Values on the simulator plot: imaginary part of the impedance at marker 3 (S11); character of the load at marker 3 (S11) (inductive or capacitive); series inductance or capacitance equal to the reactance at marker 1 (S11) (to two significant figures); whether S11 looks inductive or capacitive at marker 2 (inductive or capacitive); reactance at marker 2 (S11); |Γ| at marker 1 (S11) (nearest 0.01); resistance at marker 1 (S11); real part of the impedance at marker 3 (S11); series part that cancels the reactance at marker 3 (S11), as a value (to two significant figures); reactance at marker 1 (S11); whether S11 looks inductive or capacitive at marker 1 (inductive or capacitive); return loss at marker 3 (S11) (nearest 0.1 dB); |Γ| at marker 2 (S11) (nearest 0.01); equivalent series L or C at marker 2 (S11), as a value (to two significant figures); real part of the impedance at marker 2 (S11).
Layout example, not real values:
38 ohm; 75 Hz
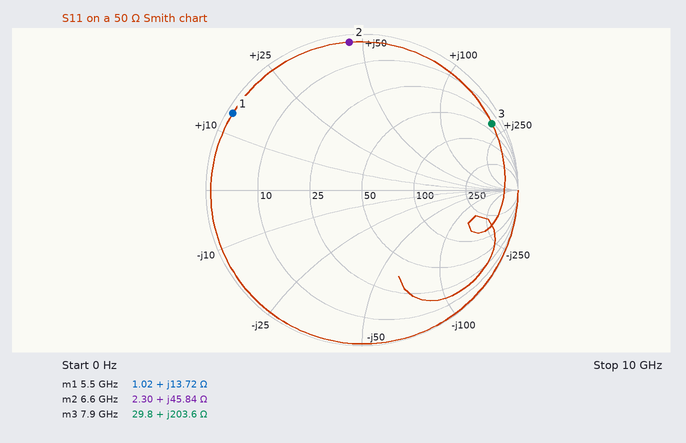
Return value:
+203.6 Ω; inductive; 400 pH; inductive; +45.84 Ω; 0.96; 1.02 Ω; 29.8 Ω; 99 fF; +13.72 Ω; inductive; 0.6 dB; 0.95; 1.1 nH; 2.30 Ω
